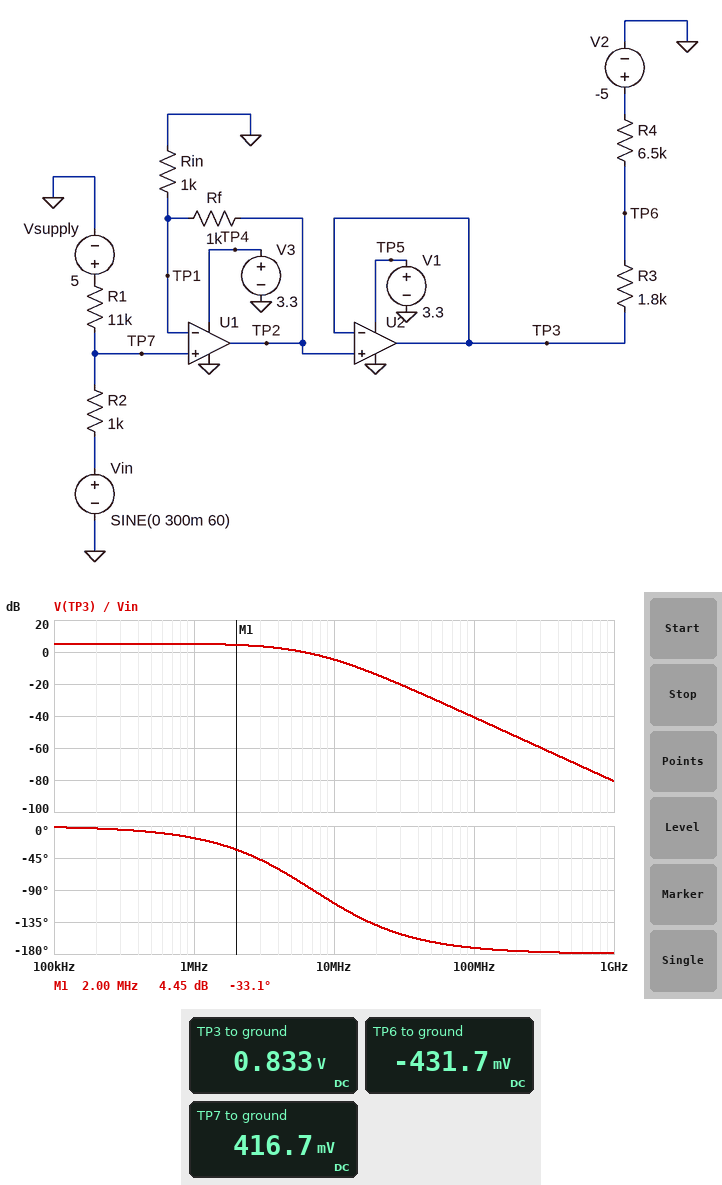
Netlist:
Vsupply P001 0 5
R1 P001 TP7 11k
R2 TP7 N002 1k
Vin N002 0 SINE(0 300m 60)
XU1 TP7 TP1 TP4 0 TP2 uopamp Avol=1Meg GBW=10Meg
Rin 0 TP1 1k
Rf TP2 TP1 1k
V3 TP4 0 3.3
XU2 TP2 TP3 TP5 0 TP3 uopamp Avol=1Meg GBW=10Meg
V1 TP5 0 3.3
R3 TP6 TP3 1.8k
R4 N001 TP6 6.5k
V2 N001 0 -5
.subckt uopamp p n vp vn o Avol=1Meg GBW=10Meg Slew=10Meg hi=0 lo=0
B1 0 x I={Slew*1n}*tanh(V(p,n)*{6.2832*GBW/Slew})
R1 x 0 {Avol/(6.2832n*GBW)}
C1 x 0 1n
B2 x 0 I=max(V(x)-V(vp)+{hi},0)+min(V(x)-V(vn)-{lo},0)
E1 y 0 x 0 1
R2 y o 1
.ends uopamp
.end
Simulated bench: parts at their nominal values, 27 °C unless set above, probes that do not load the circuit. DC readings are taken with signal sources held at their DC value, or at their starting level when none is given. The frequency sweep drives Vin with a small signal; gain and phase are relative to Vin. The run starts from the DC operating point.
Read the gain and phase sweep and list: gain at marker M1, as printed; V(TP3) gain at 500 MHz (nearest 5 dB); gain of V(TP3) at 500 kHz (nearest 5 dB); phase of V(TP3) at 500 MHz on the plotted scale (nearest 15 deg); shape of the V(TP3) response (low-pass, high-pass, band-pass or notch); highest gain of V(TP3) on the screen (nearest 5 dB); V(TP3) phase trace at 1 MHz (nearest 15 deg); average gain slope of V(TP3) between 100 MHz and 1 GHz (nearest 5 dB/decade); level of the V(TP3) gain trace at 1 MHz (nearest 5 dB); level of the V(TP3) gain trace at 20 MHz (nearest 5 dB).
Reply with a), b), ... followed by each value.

a) 4.45 dB
b) -70 dB
c) 5 dB
d) -180 deg
e) low-pass
f) 5 dB
g) -15 deg
h) -40 dB/decade
i) 5 dB
j) -15 dB
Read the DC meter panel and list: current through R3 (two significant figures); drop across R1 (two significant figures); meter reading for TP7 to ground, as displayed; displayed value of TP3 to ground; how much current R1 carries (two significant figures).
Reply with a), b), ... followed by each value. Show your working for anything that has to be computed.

a) (833 mV - (-431.7 mV)) / 1.8 kΩ = 700 µA
b) 5 V - 416.7 mV = 4.6 V
c) 416.7 mV
d) 0.833 V
e) (5 V - 416.7 mV) / 11 kΩ = 420 µA
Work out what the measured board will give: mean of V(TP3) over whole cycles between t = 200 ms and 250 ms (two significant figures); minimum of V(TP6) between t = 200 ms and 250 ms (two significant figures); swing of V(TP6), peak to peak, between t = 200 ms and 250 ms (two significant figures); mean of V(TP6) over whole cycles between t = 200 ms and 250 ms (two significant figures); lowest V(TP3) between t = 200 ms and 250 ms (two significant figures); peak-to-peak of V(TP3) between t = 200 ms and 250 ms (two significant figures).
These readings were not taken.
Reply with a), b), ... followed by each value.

a) 830 mV
b) -860 mV
c) 860 mV
d) -430 mV
e) 280 mV
f) 1.1 V
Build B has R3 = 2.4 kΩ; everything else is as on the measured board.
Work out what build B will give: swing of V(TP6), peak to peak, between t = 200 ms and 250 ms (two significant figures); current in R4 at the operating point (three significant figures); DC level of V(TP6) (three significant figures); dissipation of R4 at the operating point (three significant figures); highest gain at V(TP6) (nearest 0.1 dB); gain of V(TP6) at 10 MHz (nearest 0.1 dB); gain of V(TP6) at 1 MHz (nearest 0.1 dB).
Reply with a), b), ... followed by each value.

a) 800 mV
b) 655 µA
c) -740 mV
d) 2.79 mW
e) 2.5 dB
f) -7.5 dB
g) 2.3 dB
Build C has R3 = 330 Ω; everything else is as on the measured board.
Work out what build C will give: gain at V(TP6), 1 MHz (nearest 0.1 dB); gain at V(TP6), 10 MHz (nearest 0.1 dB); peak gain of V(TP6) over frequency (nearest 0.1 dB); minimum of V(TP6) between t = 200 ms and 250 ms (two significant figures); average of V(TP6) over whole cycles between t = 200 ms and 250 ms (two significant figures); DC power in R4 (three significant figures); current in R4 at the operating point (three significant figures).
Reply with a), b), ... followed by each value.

a) 4.6 dB
b) -5.2 dB
c) 4.8 dB
d) 28 mV
e) 550 mV
f) 4.74 mW
g) 854 µA
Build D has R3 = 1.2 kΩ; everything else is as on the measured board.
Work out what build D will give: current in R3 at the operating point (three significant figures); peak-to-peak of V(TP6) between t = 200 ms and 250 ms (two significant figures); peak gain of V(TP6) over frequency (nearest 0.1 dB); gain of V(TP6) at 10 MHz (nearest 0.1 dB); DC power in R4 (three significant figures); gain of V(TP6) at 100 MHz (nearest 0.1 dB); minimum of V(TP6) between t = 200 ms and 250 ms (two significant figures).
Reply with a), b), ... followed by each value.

a) 758 µA
b) 930 mV
c) 3.8 dB
d) -6.2 dB
e) 3.73 mW
f) -42.3 dB
g) -540 mV
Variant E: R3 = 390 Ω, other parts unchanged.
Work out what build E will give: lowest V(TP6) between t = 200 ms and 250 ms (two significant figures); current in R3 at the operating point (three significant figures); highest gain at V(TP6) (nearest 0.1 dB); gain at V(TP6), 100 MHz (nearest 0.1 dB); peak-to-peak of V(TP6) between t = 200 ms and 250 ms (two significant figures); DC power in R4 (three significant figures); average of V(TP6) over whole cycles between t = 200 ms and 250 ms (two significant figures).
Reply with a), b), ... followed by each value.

a) -16 mV
b) 847 µA
c) 4.8 dB
d) -41.3 dB
e) 1.0 V
f) 4.66 mW
g) 500 mV
